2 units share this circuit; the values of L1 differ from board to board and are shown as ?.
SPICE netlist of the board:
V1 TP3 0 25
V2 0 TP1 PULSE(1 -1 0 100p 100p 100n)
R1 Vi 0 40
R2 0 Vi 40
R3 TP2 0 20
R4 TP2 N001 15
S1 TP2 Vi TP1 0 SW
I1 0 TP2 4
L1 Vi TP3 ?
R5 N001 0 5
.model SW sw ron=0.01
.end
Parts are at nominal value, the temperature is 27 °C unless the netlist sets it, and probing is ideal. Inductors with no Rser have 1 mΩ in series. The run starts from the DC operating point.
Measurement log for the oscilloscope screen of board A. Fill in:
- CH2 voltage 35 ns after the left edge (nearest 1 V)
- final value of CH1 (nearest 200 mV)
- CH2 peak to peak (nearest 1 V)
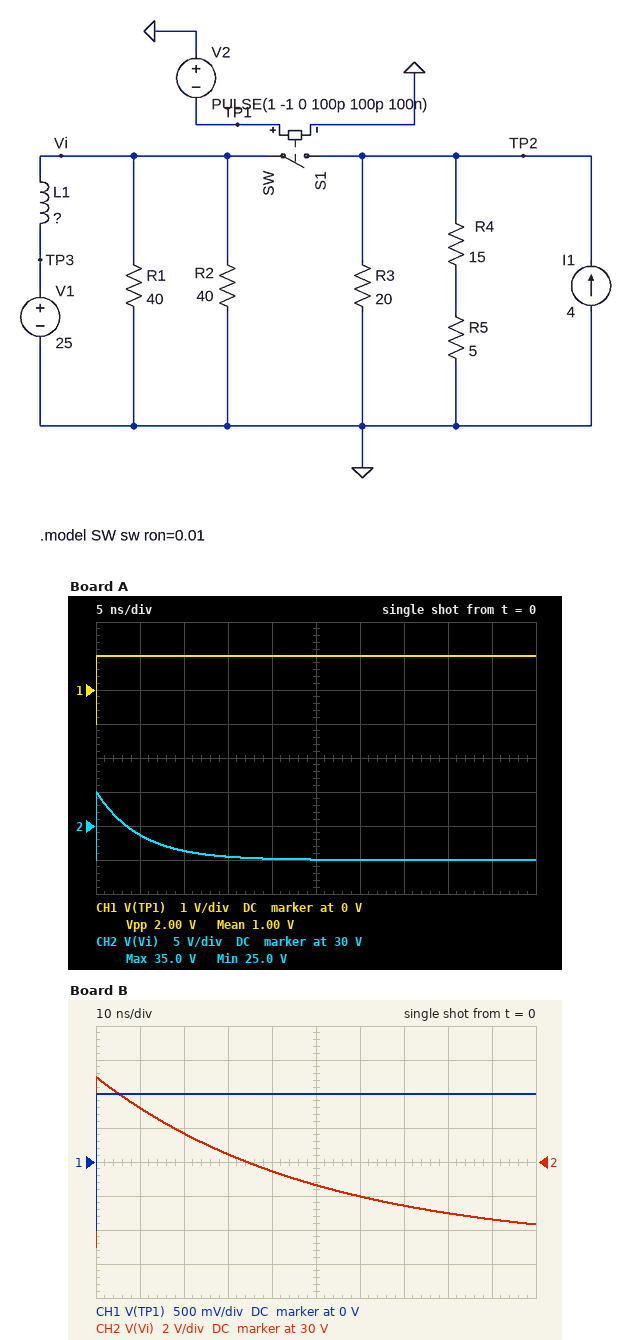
25 V
1.0 V
10 V
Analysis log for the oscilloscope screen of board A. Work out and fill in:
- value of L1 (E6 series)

33 nH
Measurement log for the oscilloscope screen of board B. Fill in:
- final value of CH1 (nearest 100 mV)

1.0 V
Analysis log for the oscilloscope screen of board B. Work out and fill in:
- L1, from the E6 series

330 nH
